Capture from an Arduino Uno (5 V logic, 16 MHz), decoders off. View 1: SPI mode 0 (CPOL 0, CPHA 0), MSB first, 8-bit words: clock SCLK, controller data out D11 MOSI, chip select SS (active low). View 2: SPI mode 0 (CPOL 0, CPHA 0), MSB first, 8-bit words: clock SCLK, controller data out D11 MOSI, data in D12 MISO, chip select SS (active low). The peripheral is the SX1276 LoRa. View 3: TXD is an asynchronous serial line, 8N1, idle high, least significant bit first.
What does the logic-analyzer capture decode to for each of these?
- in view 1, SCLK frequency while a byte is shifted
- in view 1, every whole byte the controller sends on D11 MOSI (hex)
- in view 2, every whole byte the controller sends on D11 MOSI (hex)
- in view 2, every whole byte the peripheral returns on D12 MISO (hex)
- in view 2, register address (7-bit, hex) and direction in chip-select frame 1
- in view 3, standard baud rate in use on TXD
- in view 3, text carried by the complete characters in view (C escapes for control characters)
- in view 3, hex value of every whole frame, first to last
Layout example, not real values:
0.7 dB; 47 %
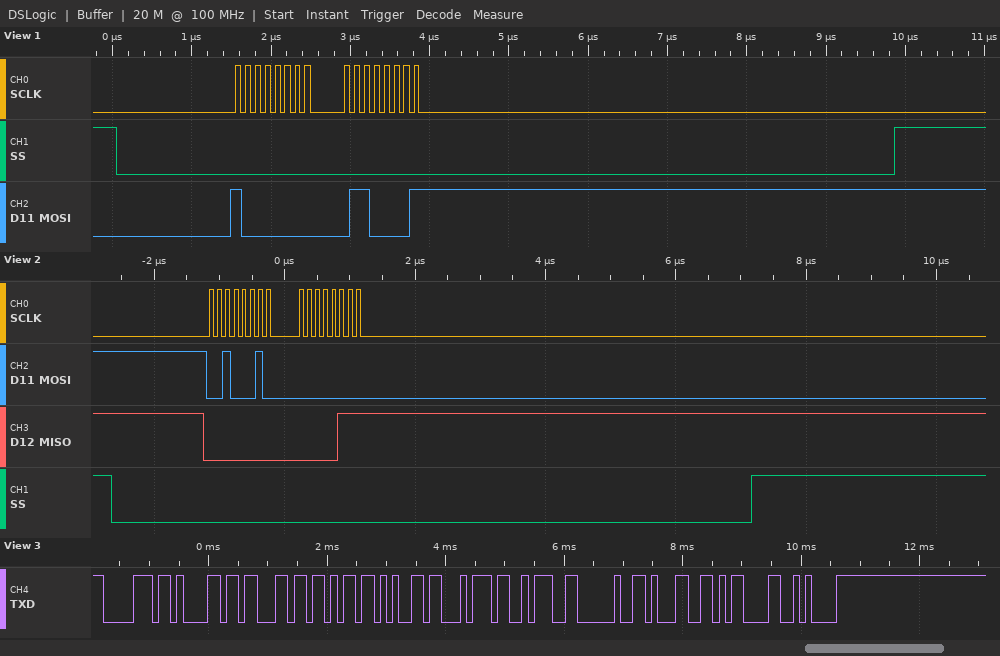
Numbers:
8 MHz; 80 61; 22 00; 00 07; 0x22 read; 9600 baud; "packet: 1\r\n"; 0x70 0x61 0x63 0x6B 0x65 0x74 0x3A 0x20 0x31 0x0D 0x0A
